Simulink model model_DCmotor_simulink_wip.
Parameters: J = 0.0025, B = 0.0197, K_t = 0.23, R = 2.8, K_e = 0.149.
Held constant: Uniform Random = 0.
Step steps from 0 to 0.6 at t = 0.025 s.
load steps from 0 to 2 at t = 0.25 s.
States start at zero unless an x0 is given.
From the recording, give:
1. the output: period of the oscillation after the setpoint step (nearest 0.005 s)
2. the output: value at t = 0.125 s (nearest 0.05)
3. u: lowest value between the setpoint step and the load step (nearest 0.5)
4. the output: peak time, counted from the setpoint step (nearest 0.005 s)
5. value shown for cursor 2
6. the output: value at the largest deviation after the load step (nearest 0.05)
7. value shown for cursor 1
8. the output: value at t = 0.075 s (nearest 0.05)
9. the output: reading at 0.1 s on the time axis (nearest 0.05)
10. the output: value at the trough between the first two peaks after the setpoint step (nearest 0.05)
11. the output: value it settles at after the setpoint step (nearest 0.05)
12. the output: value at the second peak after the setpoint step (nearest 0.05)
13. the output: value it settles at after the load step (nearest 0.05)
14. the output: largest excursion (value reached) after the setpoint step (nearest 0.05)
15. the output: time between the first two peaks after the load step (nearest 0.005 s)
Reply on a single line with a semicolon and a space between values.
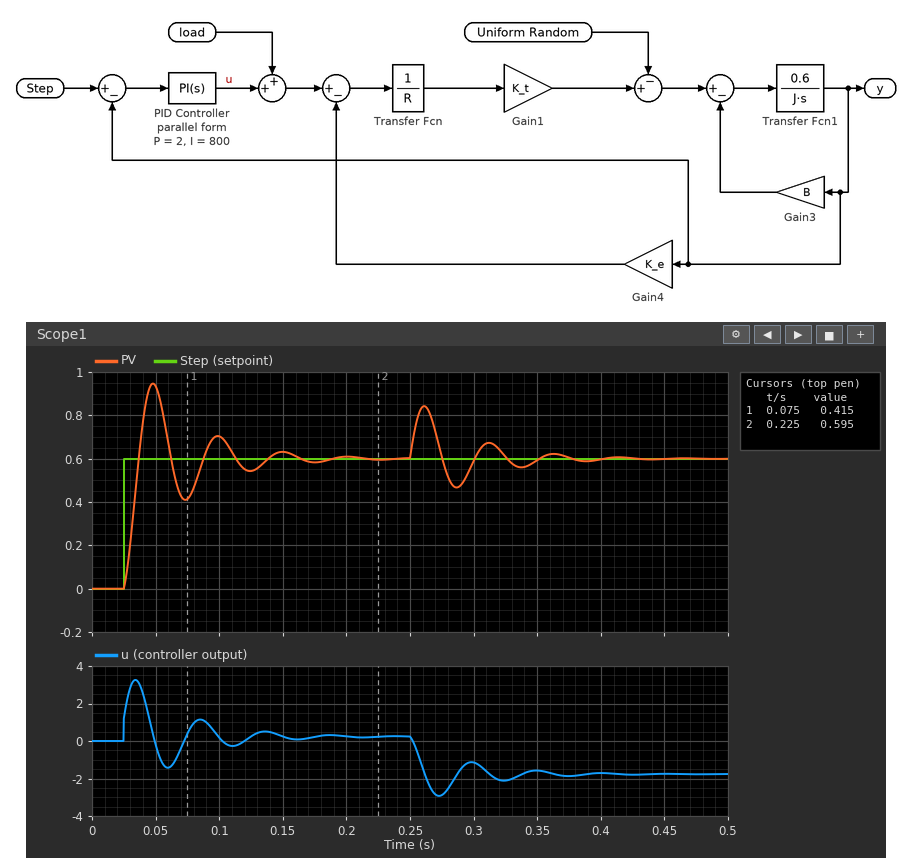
0.050 s; 0.55; -1.5; 0.025 s; 0.595; 0.85; 0.415; 0.40; 0.70; 0.40; 0.60; 0.70; 0.60; 0.95; 0.050 s
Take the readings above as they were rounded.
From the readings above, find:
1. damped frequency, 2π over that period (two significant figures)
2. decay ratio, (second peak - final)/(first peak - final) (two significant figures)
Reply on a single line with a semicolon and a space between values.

130 rad/s; 0.29
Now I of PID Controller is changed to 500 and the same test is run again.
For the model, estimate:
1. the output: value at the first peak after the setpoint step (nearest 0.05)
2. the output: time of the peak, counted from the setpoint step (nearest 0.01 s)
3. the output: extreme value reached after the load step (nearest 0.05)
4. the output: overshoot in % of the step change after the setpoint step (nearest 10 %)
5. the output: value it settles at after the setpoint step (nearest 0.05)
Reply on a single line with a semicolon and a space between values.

0.90; 0.03 s; 0.90; 50 %; 0.60
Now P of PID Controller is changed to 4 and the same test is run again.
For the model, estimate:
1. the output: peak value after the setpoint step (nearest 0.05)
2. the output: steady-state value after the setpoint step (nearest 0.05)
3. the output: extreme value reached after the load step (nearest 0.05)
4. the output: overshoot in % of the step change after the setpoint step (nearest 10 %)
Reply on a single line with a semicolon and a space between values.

0.85; 0.60; 0.80; 40 %
